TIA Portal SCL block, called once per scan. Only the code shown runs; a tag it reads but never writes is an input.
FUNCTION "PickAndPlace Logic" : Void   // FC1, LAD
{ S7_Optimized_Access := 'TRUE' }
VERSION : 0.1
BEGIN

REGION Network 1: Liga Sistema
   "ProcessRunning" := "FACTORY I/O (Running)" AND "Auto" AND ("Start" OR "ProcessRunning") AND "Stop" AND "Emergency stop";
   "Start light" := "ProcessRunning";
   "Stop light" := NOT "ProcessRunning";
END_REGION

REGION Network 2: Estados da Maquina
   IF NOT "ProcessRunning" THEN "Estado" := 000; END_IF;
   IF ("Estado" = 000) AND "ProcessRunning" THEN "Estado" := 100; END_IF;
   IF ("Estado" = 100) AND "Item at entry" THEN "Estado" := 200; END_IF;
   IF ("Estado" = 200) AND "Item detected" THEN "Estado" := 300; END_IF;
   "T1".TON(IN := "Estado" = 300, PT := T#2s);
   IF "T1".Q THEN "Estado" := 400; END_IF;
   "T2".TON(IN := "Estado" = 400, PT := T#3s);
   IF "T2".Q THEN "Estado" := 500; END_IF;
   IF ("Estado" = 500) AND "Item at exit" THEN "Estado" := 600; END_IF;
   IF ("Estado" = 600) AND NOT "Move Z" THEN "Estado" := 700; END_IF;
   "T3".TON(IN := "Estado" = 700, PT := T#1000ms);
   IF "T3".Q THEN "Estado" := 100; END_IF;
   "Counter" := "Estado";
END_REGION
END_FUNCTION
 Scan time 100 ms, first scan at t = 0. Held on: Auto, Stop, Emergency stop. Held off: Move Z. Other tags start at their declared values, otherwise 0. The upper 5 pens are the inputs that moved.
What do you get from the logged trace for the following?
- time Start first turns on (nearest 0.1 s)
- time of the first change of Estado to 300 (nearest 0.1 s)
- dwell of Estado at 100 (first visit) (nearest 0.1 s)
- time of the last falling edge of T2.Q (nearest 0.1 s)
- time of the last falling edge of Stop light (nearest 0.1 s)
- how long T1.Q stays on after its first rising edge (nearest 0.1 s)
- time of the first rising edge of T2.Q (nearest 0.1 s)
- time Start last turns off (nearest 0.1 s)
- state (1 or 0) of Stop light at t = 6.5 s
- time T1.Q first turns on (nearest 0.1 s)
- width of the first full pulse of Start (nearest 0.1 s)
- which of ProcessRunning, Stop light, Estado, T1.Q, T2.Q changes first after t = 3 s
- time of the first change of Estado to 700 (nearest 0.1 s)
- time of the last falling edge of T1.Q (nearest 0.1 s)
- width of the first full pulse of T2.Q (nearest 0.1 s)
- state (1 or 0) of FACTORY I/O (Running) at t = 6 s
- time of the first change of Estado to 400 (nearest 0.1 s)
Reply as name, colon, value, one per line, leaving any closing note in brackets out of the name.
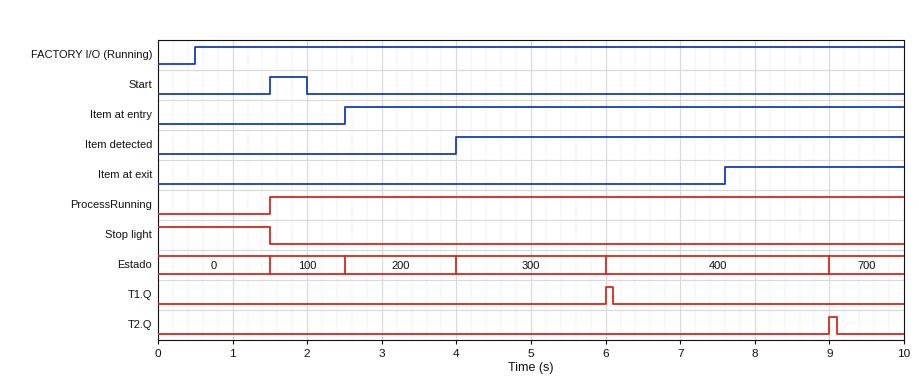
time Start first turns on: 1.5 s
time of the first change of Estado to 300: 4.0 s
dwell of Estado at 100 (first visit): 1.0 s
time of the last falling edge of T2.Q: 9.1 s
time of the last falling edge of Stop light: 1.5 s
how long T1.Q stays on after its first rising edge: 0.1 s
time of the first rising edge of T2.Q: 9.0 s
time Start last turns off: 2.0 s
state (1 or 0) of Stop light at t = 6.5 s: 0
time T1.Q first turns on: 6.0 s
width of the first full pulse of Start: 0.5 s
which of ProcessRunning, Stop light, Estado, T1.Q, T2.Q changes first after t = 3 s: Estado
time of the first change of Estado to 700: 9.0 s
time of the last falling edge of T1.Q: 6.1 s
width of the first full pulse of T2.Q: 0.1 s
state (1 or 0) of FACTORY I/O (Running) at t = 6 s: 1
time of the first change of Estado to 400: 6.0 s
